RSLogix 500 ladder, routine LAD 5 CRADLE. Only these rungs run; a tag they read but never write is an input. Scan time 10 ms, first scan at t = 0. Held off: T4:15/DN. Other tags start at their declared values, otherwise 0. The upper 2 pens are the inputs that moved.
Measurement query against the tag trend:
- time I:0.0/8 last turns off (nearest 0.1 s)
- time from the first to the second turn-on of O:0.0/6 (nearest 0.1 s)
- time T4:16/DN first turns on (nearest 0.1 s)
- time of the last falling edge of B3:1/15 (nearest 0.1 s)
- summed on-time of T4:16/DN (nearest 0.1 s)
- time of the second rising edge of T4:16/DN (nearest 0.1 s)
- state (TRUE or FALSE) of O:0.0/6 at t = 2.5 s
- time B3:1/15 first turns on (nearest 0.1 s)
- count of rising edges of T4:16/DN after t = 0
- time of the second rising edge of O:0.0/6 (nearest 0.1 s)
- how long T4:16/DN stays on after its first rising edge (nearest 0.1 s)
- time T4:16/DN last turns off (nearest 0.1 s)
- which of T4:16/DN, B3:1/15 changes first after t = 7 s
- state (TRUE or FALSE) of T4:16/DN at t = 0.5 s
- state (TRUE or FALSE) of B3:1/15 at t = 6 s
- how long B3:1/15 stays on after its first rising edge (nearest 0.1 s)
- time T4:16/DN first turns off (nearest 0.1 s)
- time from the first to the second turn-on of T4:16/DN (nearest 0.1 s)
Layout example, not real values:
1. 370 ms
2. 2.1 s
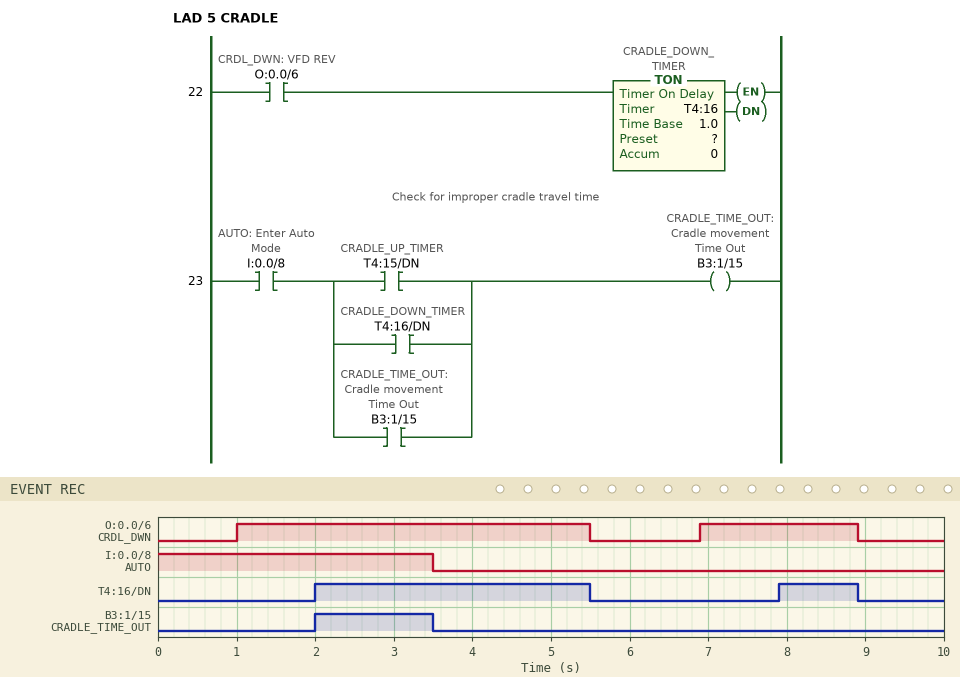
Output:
1. 3.5 s
2. 5.9 s
3. 2.0 s
4. 3.5 s
5. 4.5 s
6. 7.9 s
7. TRUE
8. 2.0 s
9. 2
10. 6.9 s
11. 3.5 s
12. 8.9 s
13. T4:16/DN
14. FALSE
15. FALSE
16. 1.5 s
17. 5.5 s
18. 5.9 s
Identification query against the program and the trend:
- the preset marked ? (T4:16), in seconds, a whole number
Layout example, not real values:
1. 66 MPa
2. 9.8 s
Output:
1. 1 s
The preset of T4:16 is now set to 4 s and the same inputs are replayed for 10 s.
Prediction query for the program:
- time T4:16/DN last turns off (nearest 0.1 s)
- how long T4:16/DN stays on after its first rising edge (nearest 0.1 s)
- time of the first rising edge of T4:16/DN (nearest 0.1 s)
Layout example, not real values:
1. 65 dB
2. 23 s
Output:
1. 5.5 s
2. 0.5 s
3. 5.0 s
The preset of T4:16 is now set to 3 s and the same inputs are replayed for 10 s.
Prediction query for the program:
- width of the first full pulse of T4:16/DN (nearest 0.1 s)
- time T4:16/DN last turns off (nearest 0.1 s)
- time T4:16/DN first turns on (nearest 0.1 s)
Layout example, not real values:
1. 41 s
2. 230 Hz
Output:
1. 1.5 s
2. 5.5 s
3. 4.0 s
